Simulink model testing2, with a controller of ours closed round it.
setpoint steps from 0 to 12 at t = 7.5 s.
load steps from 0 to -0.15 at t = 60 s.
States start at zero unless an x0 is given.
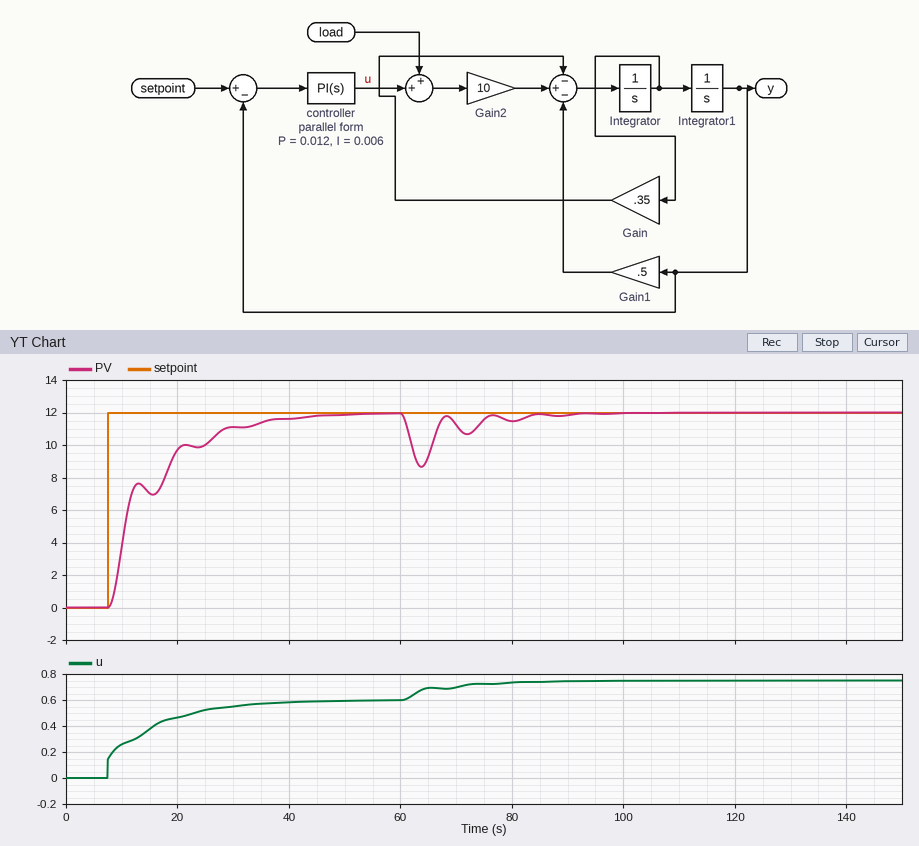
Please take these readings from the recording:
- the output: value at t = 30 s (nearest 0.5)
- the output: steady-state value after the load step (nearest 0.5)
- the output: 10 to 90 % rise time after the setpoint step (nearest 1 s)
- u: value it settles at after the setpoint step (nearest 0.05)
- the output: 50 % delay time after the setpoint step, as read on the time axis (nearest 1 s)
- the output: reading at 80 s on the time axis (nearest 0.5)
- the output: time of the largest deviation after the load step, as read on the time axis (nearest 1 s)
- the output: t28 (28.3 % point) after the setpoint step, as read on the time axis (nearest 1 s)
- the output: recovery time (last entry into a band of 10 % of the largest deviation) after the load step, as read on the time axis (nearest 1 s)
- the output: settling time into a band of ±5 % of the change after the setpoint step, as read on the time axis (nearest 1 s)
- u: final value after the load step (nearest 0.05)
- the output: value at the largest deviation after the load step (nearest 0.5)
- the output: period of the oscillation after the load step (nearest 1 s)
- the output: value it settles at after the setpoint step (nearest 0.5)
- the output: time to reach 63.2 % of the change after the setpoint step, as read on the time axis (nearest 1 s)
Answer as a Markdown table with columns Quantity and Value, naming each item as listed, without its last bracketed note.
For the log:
| Quantity | Value |
|---|---|
| the output: value at t = 30 s | 11.0 |
| the output: steady-state value after the load step | 12.0 |
| the output: 10 to 90 % rise time after the setpoint step | 19 s |
| u: value it settles at after the setpoint step | 0.60 |
| the output: 50 % delay time after the setpoint step, as read on the time axis | 11 s |
| the output: reading at 80 s on the time axis | 11.5 |
| the output: time of the largest deviation after the load step, as read on the time axis | 64 s |
| the output: t28 (28.3 % point) after the setpoint step, as read on the time axis | 10 s |
| the output: recovery time (last entry into a band of 10 % of the largest deviation) after the load step, as read on the time axis | 82 s |
| the output: settling time into a band of ±5 % of the change after the setpoint step, as read on the time axis | 35 s |
| u: final value after the load step | 0.75 |
| the output: value at the largest deviation after the load step | 8.5 |
| the output: period of the oscillation after the load step | 8 s |
| the output: value it settles at after the setpoint step | 12.0 |
| the output: time to reach 63.2 % of the change after the setpoint step, as read on the time axis | 13 s |
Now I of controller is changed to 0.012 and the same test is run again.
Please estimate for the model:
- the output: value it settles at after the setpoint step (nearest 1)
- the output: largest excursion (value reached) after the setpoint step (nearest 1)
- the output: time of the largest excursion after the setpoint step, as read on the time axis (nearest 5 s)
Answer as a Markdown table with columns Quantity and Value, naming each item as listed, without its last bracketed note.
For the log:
| Quantity | Value |
|---|---|
| the output: value it settles at after the setpoint step | 12 |
| the output: largest excursion (value reached) after the setpoint step | 13 |
| the output: time of the largest excursion after the setpoint step, as read on the time axis | 20 s |
